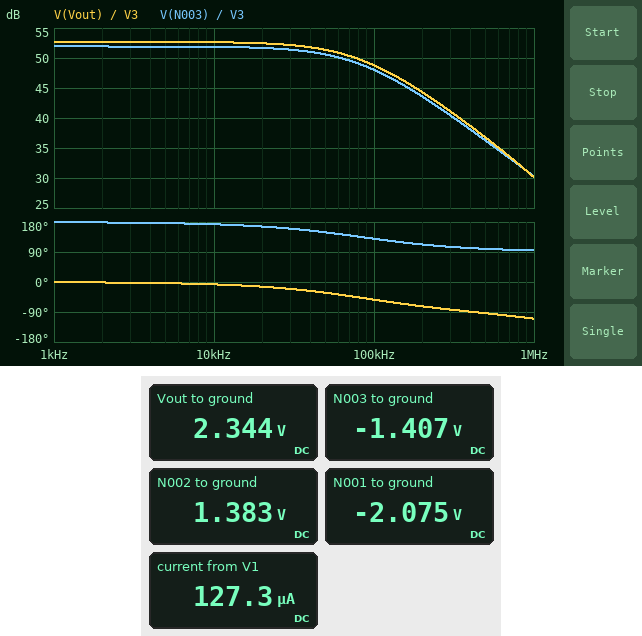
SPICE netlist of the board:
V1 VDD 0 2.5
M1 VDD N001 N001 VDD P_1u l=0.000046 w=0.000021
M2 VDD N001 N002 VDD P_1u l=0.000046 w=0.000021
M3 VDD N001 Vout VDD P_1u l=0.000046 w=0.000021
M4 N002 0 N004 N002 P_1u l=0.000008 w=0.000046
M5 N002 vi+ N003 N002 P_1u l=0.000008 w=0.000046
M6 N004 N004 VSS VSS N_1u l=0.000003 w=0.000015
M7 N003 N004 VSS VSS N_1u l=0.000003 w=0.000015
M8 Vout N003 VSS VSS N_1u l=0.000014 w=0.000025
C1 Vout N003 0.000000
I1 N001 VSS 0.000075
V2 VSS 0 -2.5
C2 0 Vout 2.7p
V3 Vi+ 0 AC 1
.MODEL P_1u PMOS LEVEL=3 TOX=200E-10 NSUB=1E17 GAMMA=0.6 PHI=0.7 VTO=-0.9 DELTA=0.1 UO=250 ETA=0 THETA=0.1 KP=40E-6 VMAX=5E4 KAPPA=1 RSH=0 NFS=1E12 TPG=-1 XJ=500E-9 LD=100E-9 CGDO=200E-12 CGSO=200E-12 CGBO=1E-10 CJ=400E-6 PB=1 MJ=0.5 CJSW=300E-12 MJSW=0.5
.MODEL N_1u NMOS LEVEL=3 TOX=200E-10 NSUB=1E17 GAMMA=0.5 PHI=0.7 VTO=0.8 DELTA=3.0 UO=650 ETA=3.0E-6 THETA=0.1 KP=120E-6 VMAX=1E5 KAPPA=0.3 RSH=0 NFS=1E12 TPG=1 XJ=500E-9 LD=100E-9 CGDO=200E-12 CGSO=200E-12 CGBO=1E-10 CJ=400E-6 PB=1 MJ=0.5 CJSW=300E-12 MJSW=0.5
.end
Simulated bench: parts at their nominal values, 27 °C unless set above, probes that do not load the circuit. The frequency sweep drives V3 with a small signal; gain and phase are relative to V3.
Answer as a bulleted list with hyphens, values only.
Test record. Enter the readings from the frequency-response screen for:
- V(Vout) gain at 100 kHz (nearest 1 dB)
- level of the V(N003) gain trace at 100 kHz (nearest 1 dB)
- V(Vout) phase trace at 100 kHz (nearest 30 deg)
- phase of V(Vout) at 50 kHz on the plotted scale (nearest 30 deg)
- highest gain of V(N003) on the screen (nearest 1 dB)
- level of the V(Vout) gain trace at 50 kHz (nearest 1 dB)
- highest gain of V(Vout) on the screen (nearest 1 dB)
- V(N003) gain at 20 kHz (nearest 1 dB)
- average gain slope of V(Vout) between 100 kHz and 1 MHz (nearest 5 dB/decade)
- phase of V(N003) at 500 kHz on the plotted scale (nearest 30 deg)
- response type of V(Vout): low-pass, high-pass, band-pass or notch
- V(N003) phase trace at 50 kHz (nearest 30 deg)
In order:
- 49 dB
- 48 dB
- -60 deg
- -30 deg
- 52 dB
- 51 dB
- 53 dB
- 52 dB
- -20 dB/decade
- 90 deg
- low-pass
- 150 deg
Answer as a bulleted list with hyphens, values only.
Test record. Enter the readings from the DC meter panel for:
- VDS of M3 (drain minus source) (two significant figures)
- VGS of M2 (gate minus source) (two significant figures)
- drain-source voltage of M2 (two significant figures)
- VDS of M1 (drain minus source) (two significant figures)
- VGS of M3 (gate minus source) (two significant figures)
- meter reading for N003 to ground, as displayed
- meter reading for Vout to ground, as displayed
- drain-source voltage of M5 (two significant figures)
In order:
- 160 mV
- -3.5 V
- 1.1 V
- 4.6 V
- -4.4 V
- -1.407 V
- 2.344 V
- 2.8 V
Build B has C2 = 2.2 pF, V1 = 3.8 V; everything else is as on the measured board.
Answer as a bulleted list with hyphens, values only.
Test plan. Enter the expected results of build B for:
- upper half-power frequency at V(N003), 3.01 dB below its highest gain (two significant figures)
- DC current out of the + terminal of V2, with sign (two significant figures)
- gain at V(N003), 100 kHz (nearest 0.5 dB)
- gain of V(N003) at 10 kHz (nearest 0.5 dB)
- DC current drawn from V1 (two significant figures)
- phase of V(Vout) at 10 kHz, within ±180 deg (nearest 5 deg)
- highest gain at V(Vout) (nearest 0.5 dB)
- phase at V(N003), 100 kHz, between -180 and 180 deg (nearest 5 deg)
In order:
- 140 kHz
- -160 µA
- 47.0 dB
- 49.0 dB
- 160 µA
- -5 deg
- 52.0 dB
- 145 deg
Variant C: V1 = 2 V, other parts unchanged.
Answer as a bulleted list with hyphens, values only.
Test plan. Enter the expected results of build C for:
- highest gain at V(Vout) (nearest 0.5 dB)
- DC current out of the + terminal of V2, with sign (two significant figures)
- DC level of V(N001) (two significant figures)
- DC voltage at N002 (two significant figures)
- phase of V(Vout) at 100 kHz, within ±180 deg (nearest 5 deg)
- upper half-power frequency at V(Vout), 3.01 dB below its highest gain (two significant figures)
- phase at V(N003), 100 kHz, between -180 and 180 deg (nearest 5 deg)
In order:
- 53.5 dB
- -110 µA
- -2.6 V
- 1.3 V
- -65 deg
- 51 kHz
- 115 deg
